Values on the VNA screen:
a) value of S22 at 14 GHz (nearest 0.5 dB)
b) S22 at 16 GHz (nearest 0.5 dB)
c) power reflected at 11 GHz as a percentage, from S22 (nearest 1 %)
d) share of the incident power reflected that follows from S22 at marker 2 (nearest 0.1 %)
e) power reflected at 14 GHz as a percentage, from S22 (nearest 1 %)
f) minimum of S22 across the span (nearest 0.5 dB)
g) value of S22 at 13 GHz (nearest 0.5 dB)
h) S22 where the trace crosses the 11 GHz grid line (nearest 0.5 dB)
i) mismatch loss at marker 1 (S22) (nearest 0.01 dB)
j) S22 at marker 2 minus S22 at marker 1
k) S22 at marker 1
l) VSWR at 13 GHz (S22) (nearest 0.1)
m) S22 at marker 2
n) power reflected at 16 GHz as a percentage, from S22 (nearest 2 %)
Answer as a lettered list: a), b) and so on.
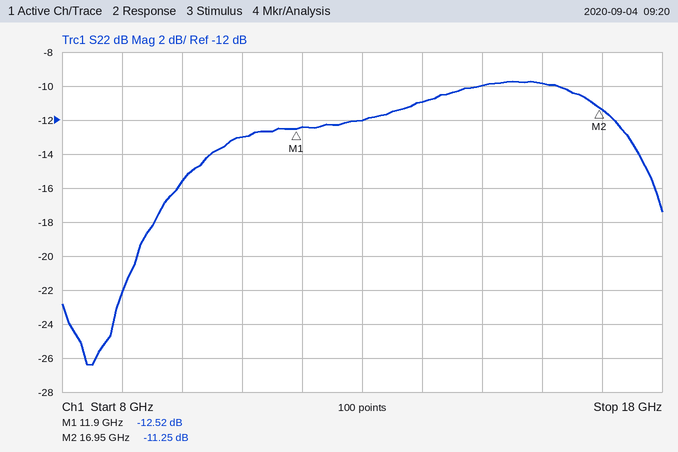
a) -11.0 dB
b) -10.0 dB
c) 5 %
d) 7.5 %
e) 8 %
f) -26.5 dB
g) -12.0 dB
h) -13.0 dB
i) 0.25 dB
j) 1.27 dB
k) -12.52 dB
l) 1.7
m) -11.25 dB
n) 10 %
